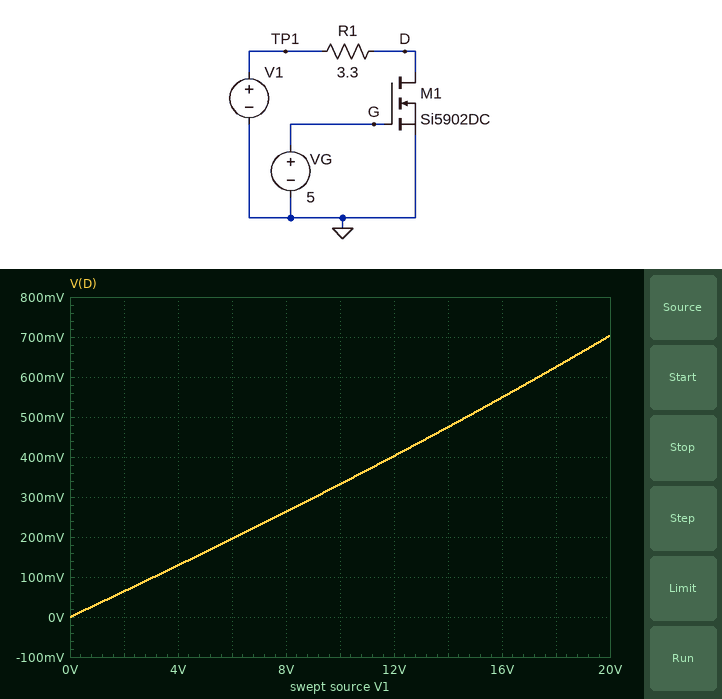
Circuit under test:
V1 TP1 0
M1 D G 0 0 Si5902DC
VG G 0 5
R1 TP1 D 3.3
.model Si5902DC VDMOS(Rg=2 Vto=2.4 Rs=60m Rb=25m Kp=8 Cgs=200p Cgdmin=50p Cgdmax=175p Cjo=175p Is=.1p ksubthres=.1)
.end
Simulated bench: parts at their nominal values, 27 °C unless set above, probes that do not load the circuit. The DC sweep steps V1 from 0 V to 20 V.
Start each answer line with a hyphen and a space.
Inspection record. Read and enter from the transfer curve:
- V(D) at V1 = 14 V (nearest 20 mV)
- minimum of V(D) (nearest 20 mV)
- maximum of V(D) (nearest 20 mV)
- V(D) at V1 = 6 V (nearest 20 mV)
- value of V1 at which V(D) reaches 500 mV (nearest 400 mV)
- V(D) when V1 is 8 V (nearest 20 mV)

- 480 mV
- 0 V
- 700 mV
- 200 mV
- 14.8 V
- 260 mV
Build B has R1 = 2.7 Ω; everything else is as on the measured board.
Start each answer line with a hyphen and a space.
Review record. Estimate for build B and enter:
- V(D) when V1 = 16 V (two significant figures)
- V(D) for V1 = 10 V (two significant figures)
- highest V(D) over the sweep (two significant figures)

- 680 mV
- 410 mV
- 880 mV
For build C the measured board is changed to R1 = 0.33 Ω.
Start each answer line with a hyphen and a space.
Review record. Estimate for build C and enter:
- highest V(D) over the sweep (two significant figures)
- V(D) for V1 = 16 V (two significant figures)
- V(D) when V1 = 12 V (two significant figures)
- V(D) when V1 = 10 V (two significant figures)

- 16 V
- 12 V
- 7.7 V
- 5.7 V
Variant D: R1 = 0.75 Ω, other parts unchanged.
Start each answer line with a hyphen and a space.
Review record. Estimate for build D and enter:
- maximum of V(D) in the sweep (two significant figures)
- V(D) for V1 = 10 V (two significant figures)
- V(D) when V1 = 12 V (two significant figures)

- 10 V
- 1.6 V
- 2.3 V
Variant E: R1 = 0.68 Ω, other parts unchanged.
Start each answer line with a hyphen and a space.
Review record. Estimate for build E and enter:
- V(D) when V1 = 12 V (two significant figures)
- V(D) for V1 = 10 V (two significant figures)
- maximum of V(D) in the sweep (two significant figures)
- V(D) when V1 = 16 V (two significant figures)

- 3.1 V
- 1.9 V
- 11 V
- 7.1 V
